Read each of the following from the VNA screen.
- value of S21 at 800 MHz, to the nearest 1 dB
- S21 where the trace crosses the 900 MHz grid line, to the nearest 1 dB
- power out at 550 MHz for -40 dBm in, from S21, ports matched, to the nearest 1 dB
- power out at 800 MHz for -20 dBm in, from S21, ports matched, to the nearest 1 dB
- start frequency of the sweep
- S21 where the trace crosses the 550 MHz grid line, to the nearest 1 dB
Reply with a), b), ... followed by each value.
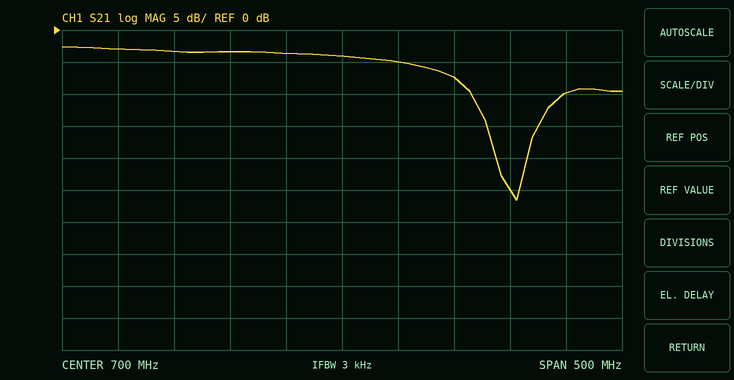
a) -7 dB
b) -10 dB
c) -43 dBm
d) -27 dBm
e) 450 MHz
f) -3 dB
